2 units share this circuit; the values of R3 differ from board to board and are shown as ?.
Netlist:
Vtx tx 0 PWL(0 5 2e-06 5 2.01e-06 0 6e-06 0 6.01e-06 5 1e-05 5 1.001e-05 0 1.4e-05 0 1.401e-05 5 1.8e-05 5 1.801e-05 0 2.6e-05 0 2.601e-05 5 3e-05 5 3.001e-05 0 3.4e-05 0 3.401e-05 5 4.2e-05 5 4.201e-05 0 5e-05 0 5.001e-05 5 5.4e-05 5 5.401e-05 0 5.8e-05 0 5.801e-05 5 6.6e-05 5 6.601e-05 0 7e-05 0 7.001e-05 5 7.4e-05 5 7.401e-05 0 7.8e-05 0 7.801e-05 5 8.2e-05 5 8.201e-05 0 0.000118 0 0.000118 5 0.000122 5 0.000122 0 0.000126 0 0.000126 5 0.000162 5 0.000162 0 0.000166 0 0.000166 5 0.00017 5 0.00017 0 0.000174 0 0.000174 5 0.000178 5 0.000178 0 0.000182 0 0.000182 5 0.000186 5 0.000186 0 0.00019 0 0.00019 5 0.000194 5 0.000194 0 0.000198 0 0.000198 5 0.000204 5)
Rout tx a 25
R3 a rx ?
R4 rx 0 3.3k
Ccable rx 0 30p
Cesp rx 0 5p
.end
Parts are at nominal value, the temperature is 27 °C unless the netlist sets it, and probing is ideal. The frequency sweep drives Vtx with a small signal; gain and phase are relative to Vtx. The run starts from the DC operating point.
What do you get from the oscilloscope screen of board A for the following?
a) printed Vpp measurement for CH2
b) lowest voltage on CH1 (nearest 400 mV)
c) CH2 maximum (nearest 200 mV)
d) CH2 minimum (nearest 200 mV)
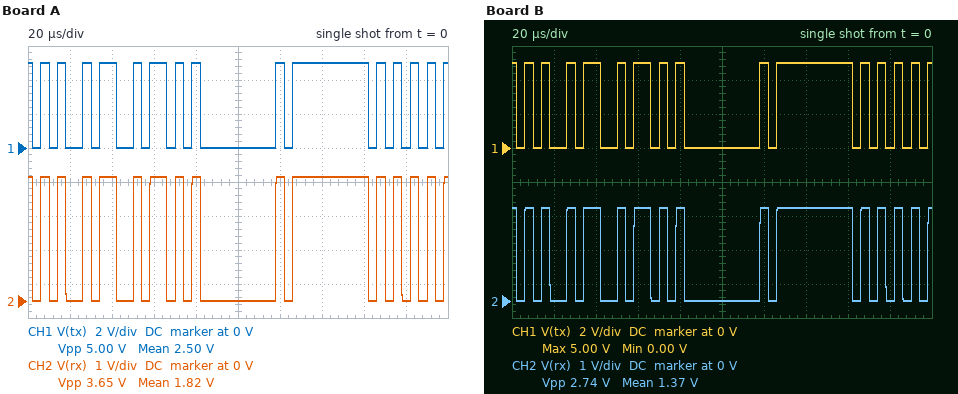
3.65 V
0 V
3.6 V
0 V
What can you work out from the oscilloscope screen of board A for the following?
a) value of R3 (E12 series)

1.2 kΩ
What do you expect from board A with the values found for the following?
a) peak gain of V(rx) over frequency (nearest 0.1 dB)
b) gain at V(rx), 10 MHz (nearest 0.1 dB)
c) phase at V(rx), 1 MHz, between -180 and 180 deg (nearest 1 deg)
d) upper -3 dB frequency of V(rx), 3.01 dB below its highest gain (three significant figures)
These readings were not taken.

-2.7 dB
-9.6 dB
-11 deg
5.09 MHz
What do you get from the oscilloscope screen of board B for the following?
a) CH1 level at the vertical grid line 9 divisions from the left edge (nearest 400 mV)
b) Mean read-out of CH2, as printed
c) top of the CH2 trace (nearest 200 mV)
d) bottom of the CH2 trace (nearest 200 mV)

0 V
1.37 V
2.8 V
0 V
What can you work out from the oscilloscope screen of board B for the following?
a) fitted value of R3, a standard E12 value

2.7 kΩ
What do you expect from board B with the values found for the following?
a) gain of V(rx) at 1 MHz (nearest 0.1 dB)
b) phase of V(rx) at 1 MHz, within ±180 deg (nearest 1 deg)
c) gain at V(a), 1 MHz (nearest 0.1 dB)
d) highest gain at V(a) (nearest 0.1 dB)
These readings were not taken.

-5.7 dB
-18 deg
0 dB
0 dB
